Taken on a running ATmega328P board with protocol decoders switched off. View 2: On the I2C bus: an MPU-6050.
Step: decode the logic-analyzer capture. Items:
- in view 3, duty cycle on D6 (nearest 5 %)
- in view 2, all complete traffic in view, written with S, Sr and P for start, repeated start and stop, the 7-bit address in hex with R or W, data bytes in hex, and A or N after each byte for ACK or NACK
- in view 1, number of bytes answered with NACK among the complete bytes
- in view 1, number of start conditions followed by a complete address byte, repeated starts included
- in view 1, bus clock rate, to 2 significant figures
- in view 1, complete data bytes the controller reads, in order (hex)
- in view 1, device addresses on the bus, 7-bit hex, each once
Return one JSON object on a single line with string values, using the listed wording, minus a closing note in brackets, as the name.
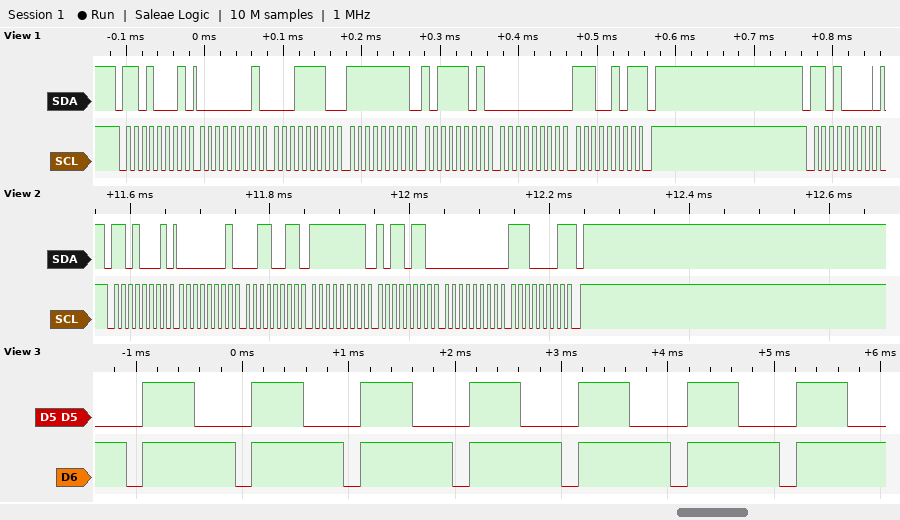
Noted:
{"in view 3, duty cycle on D6": "85 %", "in view 2, all complete traffic in view, written with S, Sr and P for start, repeated start and stop, the 7-bit address in hex with R or W, data bytes in hex, and A or N after each byte for ACK or NACK": "S 68R A 01 A 33 A FF A B6 A 00 A E1 N P", "in view 1, number of bytes answered with NACK among the complete bytes": "1", "in view 1, number of start conditions followed by a complete address byte, repeated starts included": "2", "in view 1, bus clock rate, to 2 significant figures": "100 kHz", "in view 1, complete data bytes the controller reads, in order": "01 1E FF BD 00 E5", "in view 1, device addresses on the bus, 7-bit hex, each once": "0x68"}
